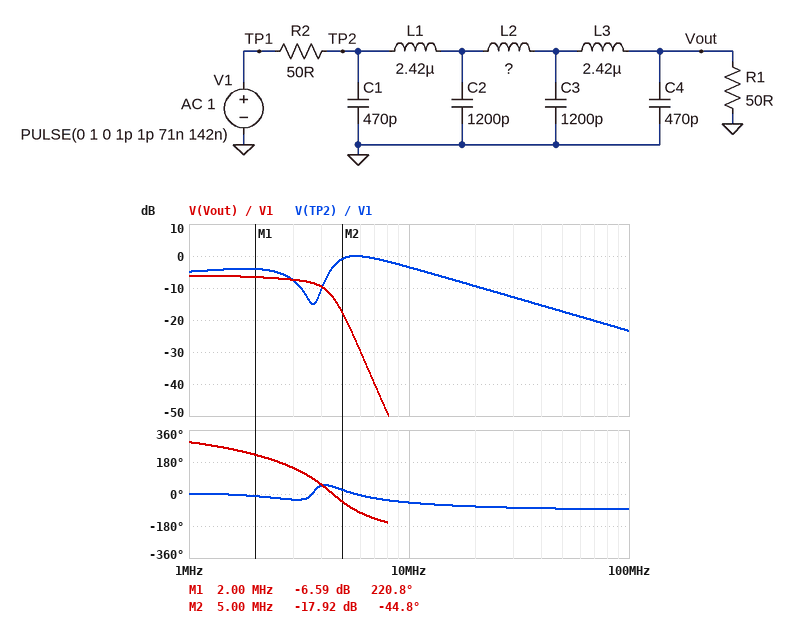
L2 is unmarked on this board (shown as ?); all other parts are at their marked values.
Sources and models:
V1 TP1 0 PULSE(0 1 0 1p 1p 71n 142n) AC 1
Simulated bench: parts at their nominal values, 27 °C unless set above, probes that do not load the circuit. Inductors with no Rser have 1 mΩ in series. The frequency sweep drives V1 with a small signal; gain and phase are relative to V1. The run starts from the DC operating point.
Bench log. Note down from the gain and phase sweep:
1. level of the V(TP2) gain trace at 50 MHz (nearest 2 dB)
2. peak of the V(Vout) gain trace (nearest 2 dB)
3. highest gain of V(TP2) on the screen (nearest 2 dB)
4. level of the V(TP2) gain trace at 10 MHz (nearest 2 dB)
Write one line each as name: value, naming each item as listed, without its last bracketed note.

level of the V(TP2) gain trace at 50 MHz: -18 dB
peak of the V(Vout) gain trace: -6 dB
highest gain of V(TP2) on the screen: 0 dB
level of the V(TP2) gain trace at 10 MHz: -4 dB
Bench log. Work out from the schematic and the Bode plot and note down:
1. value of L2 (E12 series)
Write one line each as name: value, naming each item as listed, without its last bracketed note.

value of L2: 5.6 µH
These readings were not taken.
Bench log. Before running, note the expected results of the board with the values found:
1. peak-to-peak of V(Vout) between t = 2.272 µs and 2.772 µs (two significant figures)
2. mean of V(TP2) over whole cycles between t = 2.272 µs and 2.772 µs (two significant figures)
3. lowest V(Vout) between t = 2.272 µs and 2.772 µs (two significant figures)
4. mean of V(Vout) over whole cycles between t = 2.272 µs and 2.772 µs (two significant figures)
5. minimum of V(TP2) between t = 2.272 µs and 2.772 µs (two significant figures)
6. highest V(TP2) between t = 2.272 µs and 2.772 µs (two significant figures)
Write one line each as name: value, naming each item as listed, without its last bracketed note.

peak-to-peak of V(Vout) between t = 2.272 µs and 2.772 µs: 12 mV
mean of V(TP2) over whole cycles between t = 2.272 µs and 2.772 µs: 250 mV
lowest V(Vout) between t = 2.272 µs and 2.772 µs: 240 mV
mean of V(Vout) over whole cycles between t = 2.272 µs and 2.772 µs: 250 mV
minimum of V(TP2) between t = 2.272 µs and 2.772 µs: -280 mV
highest V(TP2) between t = 2.272 µs and 2.772 µs: 780 mV
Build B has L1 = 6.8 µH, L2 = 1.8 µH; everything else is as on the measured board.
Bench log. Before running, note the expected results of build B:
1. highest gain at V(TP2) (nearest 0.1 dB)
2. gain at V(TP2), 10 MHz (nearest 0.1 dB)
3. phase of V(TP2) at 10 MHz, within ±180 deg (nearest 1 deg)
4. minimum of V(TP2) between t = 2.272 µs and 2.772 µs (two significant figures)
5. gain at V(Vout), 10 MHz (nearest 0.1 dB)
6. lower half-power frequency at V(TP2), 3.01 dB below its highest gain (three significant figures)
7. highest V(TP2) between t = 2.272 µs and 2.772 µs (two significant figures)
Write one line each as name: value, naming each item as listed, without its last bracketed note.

highest gain at V(TP2): -0.6 dB
gain at V(TP2), 10 MHz: -4.5 dB
phase of V(TP2) at 10 MHz, within ±180 deg: -54 deg
minimum of V(TP2) between t = 2.272 µs and 2.772 µs: -200 mV
gain at V(Vout), 10 MHz: -62.9 dB
lower half-power frequency at V(TP2), 3.01 dB below its highest gain: 1.63 MHz
highest V(TP2) between t = 2.272 µs and 2.772 µs: 700 mV
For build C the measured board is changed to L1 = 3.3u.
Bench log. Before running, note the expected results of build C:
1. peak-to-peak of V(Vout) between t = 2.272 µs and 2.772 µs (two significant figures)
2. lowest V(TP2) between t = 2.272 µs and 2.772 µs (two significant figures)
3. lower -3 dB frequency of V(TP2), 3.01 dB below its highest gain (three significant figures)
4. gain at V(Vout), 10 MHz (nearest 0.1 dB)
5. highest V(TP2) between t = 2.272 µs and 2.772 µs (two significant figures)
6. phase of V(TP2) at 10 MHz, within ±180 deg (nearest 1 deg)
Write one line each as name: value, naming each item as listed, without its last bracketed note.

peak-to-peak of V(Vout) between t = 2.272 µs and 2.772 µs: 7.6 mV
lowest V(TP2) between t = 2.272 µs and 2.772 µs: -230 mV
lower -3 dB frequency of V(TP2), 3.01 dB below its highest gain: 4.00 MHz
gain at V(Vout), 10 MHz: -67.4 dB
highest V(TP2) between t = 2.272 µs and 2.772 µs: 730 mV
phase of V(TP2) at 10 MHz, within ±180 deg: -51 deg
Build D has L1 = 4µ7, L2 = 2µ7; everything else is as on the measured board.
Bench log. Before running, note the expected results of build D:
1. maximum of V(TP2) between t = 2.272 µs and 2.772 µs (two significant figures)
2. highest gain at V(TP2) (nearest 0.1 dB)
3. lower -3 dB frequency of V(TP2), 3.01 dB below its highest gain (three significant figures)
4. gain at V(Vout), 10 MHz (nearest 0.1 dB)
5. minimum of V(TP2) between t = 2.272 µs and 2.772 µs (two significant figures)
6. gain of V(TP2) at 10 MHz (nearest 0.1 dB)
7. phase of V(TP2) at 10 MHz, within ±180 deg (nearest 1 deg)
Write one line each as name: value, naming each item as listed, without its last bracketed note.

maximum of V(TP2) between t = 2.272 µs and 2.772 µs: 710 mV
highest gain at V(TP2): -0.7 dB
lower -3 dB frequency of V(TP2), 3.01 dB below its highest gain: 2.31 MHz
gain at V(Vout), 10 MHz: -63.8 dB
minimum of V(TP2) between t = 2.272 µs and 2.772 µs: -210 mV
gain of V(TP2) at 10 MHz: -4.3 dB
phase of V(TP2) at 10 MHz, within ±180 deg: -52 deg
